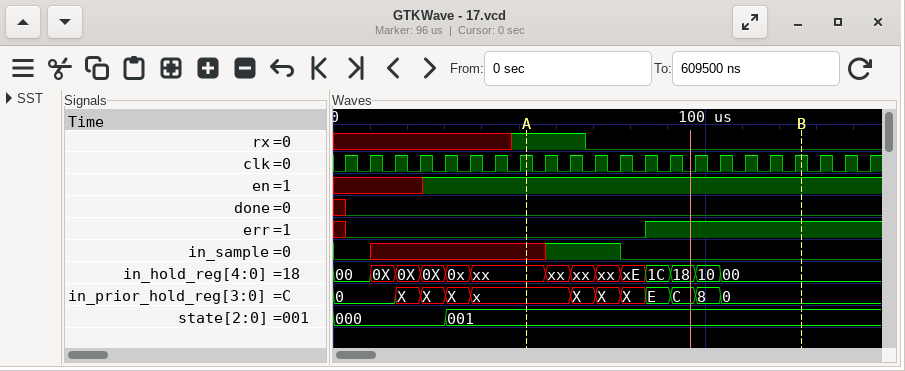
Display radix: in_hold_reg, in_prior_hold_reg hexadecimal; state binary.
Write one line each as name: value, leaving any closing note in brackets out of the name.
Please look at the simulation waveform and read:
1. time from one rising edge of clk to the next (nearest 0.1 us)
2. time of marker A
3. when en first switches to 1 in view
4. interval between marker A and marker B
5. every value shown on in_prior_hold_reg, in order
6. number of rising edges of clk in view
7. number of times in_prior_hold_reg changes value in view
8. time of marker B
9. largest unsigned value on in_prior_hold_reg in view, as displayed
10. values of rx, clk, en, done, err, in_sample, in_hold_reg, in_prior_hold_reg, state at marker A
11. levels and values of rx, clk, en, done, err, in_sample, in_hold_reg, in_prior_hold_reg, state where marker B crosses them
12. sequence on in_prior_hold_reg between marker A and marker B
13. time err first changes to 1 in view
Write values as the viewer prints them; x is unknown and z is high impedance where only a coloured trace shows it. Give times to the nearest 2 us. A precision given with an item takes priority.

time from one rising edge of clk to the next: 6.7 us
time of marker A: 52 us
when en first switches to 1 in view: 24 us
interval between marker A and marker B: 74 us
every value shown on in_prior_hold_reg, in order: 0, X, X, X, x, X, X, X, E, C, 8, 0
number of rising edges of clk in view: 22
number of times in_prior_hold_reg changes value in view: 11
time of marker B: 126 us
largest unsigned value on in_prior_hold_reg in view, as displayed: E
values of rx, clk, en, done, err, in_sample, in_hold_reg, in_prior_hold_reg, state at marker A: rx=1, clk=1, en=1, done=0, err=0, in_sample=x, in_hold_reg=xx, in_prior_hold_reg=x, state=001
levels and values of rx, clk, en, done, err, in_sample, in_hold_reg, in_prior_hold_reg, state where marker B crosses them: rx=0, clk=1, en=1, done=0, err=1, in_sample=0, in_hold_reg=00, in_prior_hold_reg=0, state=001
sequence on in_prior_hold_reg between marker A and marker B: x, X, X, X, E, C, 8, 0
time err first changes to 1 in view: 84 us
